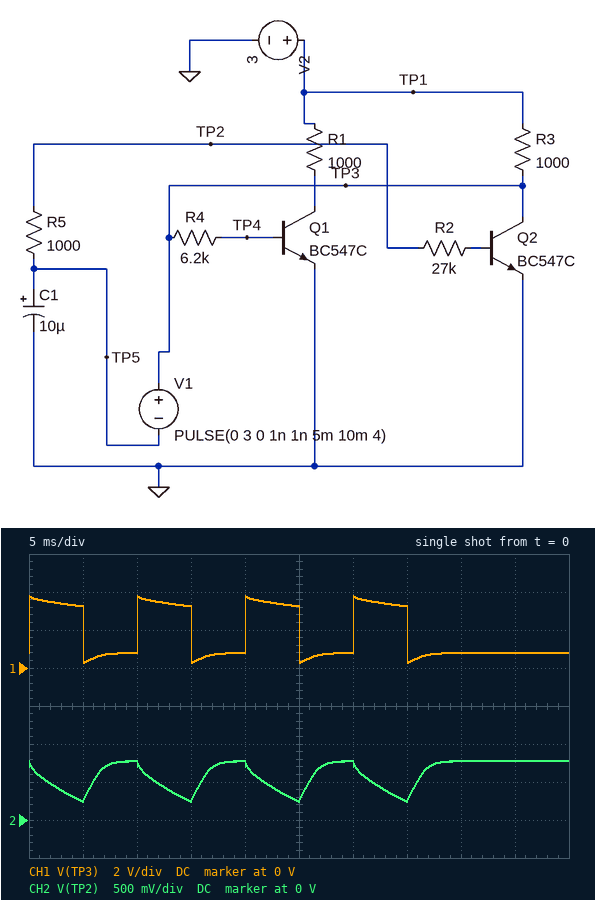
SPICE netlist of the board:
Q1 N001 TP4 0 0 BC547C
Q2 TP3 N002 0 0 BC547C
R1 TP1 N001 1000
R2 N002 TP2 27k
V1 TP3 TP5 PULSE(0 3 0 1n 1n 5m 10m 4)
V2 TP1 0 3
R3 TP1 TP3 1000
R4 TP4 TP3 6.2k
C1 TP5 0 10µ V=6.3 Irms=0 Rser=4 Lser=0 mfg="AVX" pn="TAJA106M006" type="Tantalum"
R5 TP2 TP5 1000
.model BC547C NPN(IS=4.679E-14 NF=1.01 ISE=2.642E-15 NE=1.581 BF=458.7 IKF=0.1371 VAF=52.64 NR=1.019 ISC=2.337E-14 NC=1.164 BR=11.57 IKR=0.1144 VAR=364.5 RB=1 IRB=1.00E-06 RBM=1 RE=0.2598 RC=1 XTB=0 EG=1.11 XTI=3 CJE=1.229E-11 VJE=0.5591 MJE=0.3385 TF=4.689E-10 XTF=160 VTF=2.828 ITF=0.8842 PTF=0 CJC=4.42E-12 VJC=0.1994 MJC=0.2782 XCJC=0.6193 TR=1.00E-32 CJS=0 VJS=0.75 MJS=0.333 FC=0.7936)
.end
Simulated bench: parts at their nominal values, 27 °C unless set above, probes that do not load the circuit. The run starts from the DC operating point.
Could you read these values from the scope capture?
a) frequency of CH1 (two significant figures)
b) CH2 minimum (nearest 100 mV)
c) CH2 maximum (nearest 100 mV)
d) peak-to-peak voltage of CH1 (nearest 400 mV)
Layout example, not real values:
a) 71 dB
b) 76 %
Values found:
a) 100 Hz
b) 200 mV
c) 800 mV
d) 3.6 V
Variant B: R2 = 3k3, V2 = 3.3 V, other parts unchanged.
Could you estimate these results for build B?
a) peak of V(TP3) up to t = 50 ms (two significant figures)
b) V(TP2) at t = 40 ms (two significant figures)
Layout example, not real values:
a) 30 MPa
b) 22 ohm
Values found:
a) 3.7 V
b) 670 mV
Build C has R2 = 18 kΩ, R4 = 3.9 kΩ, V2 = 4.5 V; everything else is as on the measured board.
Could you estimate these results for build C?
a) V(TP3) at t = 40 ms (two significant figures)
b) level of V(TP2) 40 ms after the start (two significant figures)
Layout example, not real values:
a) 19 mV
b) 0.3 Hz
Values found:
a) 810 mV
b) 800 mV
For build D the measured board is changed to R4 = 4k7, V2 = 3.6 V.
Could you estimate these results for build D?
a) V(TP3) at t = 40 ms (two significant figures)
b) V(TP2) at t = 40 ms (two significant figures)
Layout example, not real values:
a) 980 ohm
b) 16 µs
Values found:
a) 820 mV
b) 810 mV
